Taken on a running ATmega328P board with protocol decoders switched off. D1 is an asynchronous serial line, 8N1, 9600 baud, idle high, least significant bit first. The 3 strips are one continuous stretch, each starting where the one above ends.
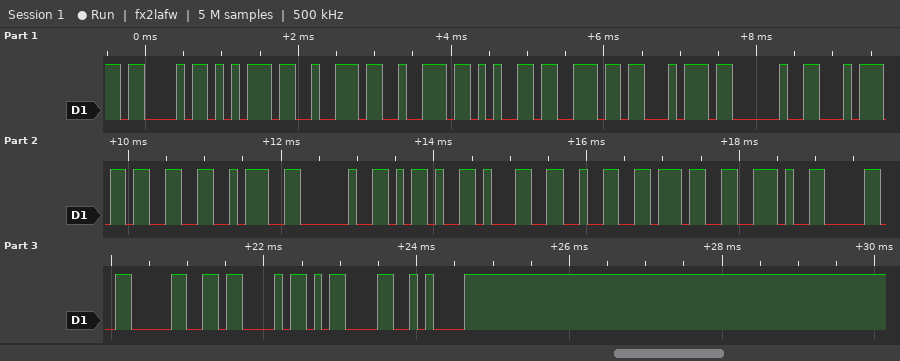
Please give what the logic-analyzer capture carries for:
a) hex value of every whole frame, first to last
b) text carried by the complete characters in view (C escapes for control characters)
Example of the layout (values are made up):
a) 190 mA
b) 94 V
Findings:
a) 43 75 72 72 65 6E 74 20 74 33 3A 20 2D 31 32 37 2E 30 30 43 0D 0A
b) "Current t3: -127.00C\r\n"
